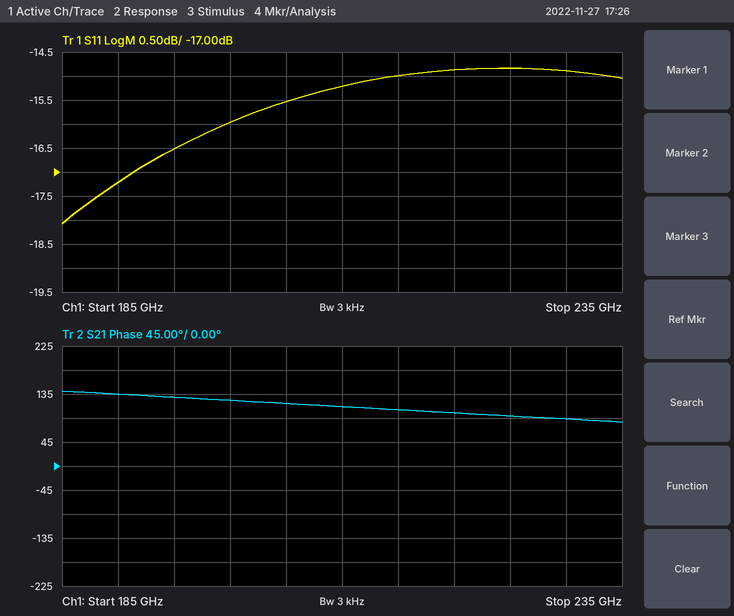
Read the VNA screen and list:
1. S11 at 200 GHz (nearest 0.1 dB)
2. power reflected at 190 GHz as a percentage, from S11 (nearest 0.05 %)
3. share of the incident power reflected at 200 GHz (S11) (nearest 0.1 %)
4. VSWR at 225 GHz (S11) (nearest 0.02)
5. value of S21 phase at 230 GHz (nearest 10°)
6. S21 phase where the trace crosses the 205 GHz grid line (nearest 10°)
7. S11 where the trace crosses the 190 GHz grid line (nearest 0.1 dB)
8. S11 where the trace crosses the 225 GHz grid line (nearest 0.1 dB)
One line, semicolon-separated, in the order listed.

-16.0 dB; 1.90 %; 2.5 %; 1.44; 90°; 120°; -17.2 dB; -14.8 dB
